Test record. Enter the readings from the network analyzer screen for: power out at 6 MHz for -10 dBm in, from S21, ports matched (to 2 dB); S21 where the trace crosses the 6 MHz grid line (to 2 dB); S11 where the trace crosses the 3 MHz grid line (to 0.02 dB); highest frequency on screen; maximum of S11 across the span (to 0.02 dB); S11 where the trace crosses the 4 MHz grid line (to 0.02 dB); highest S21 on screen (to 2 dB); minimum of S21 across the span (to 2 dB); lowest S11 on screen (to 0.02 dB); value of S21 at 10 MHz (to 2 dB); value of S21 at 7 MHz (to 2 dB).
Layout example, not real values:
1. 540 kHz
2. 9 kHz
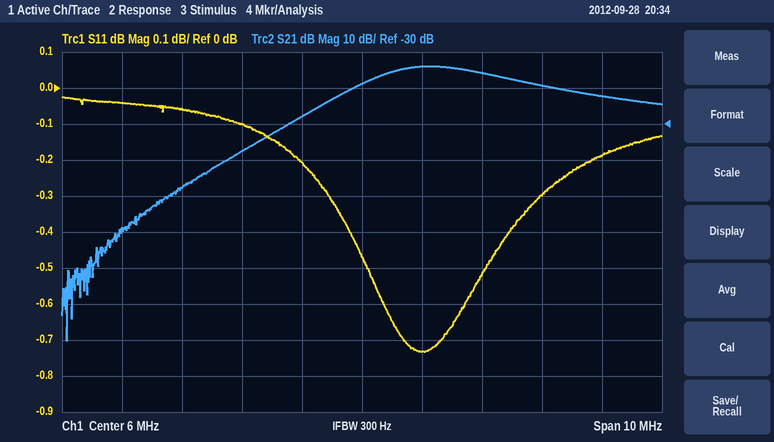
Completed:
1. -28 dBm
2. -18 dB
3. -0.06 dB
4. 11 MHz
5. -0.02 dB
6. -0.10 dB
7. -14 dB
8. -90 dB
9. -0.74 dB
10. -22 dB
11. -14 dB
